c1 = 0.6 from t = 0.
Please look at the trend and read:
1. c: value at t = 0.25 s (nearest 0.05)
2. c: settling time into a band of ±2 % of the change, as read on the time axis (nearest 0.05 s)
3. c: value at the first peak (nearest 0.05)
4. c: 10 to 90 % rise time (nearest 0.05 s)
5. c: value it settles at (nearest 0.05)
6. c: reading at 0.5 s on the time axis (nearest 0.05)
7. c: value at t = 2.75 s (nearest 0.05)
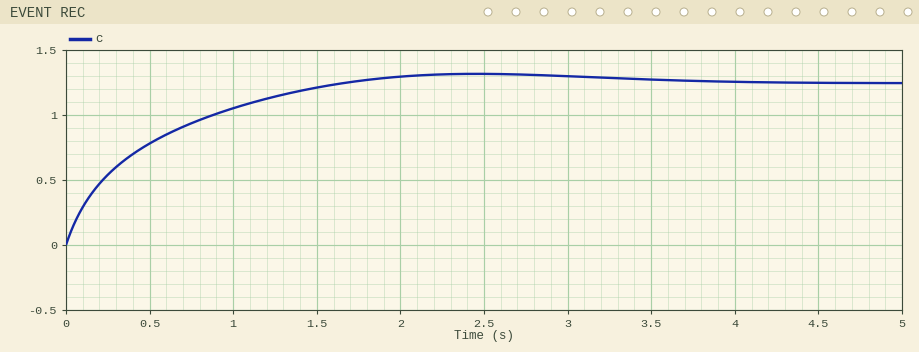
0.55
3.50 s
1.30
1.15 s
1.25
0.80
1.30
